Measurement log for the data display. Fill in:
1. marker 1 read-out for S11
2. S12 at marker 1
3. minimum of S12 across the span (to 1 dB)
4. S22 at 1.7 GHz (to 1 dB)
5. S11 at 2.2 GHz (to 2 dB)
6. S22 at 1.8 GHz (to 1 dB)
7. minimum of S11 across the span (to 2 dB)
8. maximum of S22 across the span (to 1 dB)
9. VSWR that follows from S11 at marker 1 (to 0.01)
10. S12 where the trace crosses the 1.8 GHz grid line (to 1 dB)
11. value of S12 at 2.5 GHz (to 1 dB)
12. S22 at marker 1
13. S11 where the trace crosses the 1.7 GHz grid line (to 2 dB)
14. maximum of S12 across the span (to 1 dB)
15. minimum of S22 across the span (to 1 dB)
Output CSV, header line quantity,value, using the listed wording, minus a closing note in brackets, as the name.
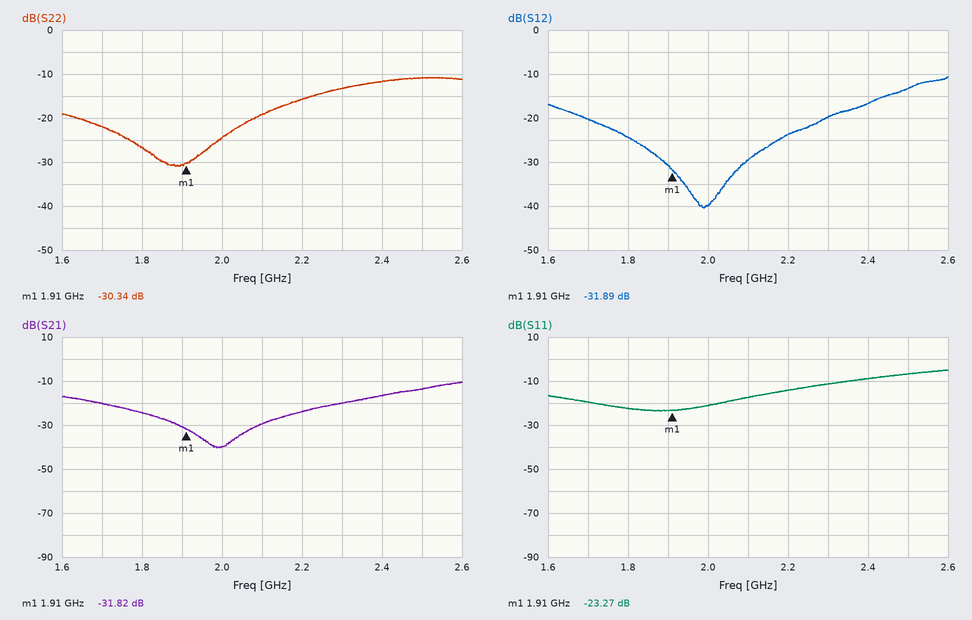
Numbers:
quantity,value
marker 1 read-out for S11,-23.27 dB
S12 at marker 1,-31.89 dB
minimum of S12 across the span,-40 dB
S22 at 1.7 GHz,-22 dB
S11 at 2.2 GHz,-14 dB
S22 at 1.8 GHz,-27 dB
minimum of S11 across the span,-24 dB
maximum of S22 across the span,-11 dB
VSWR that follows from S11 at marker 1,1.15
S12 where the trace crosses the 1.8 GHz grid line,-24 dB
value of S12 at 2.5 GHz,-13 dB
S22 at marker 1,-30.34 dB
S11 where the trace crosses the 1.7 GHz grid line,-20 dB
maximum of S12 across the span,-11 dB
minimum of S22 across the span,-31 dB
